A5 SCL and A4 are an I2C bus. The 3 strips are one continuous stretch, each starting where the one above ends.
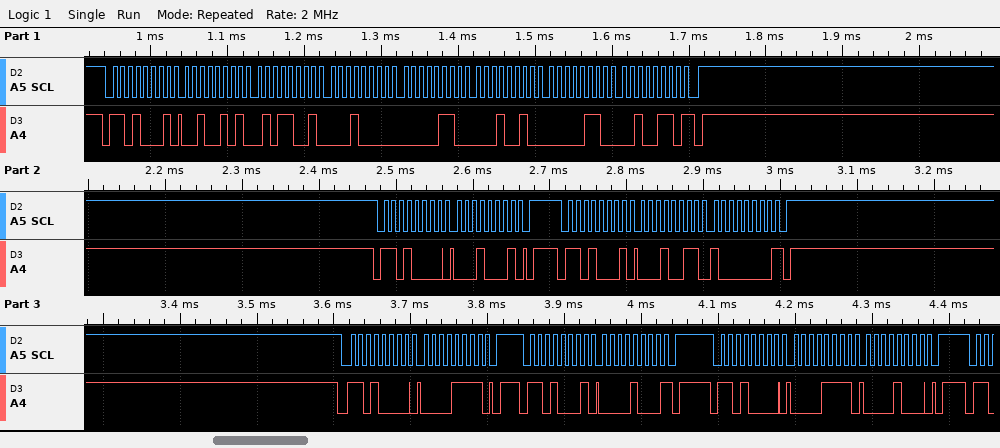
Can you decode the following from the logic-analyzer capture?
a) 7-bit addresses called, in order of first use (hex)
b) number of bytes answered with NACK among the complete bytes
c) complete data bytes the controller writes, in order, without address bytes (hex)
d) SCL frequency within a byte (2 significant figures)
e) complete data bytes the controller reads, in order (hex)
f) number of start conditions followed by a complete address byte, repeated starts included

0x68
3
11 0F 0F 08
100 kHz
25 59 10 06 12 06 26 13 80 08
6
